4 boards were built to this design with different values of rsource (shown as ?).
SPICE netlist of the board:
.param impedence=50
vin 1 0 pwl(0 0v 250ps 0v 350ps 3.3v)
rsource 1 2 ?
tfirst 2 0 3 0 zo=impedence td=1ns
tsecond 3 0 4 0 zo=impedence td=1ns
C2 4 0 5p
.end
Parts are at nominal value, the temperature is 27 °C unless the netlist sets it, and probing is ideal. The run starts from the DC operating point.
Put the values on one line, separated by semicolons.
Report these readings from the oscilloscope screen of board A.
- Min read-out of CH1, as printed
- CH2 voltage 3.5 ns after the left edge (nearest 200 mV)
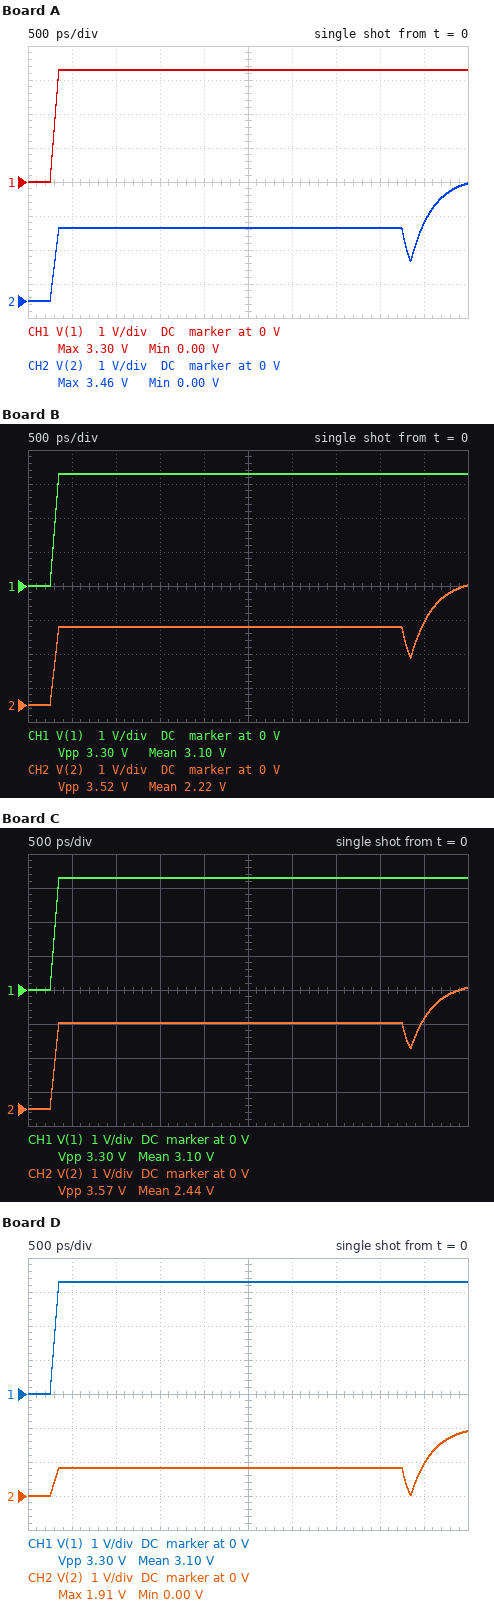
0.00 V; 2.2 V
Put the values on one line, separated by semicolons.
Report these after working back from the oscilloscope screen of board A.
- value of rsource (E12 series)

27 Ω
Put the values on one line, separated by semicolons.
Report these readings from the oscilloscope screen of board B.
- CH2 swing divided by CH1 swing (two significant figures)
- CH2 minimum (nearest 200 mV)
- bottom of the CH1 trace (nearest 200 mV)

1.1; 0 V; 0 V
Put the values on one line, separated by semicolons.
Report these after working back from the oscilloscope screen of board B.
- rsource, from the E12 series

22 Ω
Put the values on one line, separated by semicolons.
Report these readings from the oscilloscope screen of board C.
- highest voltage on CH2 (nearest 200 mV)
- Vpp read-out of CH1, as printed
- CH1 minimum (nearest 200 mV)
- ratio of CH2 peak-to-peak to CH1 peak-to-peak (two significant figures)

3.6 V; 3.30 V; 0 V; 1.1
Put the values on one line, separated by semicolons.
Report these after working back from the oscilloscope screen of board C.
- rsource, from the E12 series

15 Ω
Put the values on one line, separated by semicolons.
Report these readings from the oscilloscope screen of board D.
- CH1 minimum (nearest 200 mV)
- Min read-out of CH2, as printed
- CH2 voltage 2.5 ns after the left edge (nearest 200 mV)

0 V; 0.00 V; 800 mV
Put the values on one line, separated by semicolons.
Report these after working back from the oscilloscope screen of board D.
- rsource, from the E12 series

150 Ω
